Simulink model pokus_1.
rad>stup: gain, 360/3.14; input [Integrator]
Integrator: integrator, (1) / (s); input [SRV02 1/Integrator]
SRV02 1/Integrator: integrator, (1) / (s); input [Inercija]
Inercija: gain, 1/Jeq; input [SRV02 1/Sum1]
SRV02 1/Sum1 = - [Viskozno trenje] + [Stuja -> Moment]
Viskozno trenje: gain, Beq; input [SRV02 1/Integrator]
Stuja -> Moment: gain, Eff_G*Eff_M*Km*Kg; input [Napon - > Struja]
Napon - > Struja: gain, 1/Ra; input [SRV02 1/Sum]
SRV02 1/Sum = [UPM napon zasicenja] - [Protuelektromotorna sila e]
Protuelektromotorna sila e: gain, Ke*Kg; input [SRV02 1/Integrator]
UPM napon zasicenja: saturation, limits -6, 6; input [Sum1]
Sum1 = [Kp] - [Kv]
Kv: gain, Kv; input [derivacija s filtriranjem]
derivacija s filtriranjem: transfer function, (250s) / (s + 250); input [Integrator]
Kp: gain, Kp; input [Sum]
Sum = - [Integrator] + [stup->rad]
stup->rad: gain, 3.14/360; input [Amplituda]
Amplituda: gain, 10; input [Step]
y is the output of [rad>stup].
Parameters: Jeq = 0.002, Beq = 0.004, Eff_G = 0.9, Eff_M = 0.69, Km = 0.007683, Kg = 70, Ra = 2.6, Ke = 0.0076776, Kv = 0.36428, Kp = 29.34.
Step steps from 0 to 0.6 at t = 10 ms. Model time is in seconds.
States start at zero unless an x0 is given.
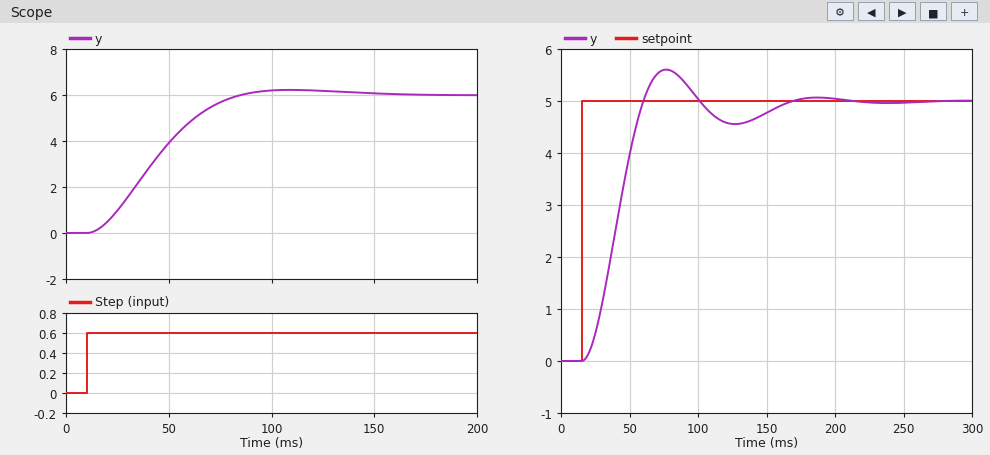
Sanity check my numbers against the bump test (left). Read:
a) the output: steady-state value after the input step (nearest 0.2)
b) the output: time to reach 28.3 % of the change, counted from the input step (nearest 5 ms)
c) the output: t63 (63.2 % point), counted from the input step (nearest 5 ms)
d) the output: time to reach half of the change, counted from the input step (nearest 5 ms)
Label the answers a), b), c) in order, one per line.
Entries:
a) 6.0
b) 20 ms
c) 40 ms
d) 30 ms
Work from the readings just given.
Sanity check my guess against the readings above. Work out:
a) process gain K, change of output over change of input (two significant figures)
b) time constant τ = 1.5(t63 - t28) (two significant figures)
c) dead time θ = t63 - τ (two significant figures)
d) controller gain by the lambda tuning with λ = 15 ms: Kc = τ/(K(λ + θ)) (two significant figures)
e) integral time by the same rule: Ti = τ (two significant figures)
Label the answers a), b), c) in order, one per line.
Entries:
a) 10
b) 30 ms
c) 10 ms
d) 0.12
e) 30 ms
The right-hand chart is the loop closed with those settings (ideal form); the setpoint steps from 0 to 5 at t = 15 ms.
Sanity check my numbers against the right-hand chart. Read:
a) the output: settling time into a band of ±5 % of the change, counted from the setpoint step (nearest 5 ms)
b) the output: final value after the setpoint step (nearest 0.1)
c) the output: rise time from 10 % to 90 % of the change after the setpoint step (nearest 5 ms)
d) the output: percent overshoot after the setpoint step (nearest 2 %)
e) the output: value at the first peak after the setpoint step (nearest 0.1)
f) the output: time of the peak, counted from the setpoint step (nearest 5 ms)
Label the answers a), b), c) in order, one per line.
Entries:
a) 135 ms
b) 5.0
c) 30 ms
d) 12 %
e) 5.6
f) 60 ms
